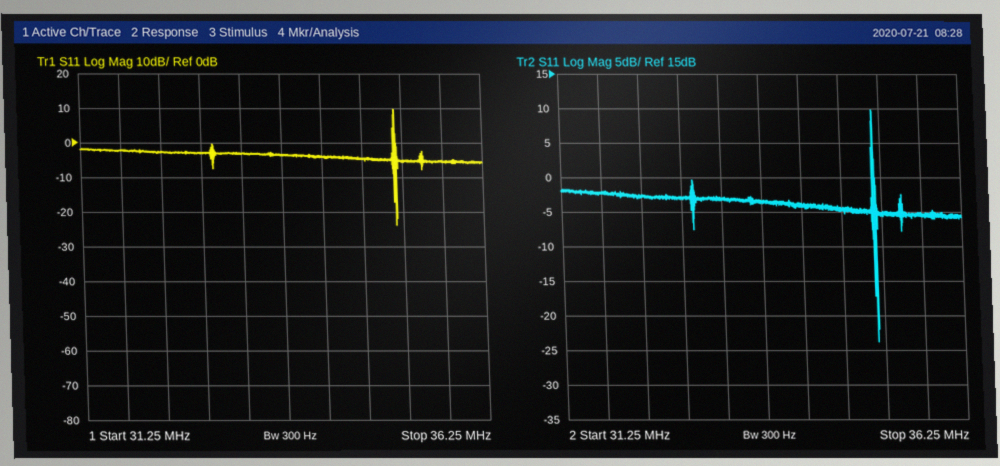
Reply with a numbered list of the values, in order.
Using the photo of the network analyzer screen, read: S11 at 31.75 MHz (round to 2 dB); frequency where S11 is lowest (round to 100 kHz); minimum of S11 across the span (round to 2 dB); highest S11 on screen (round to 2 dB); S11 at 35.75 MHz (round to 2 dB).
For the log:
1. -2 dB
2. 35.2 MHz
3. -24 dB
4. 10 dB
5. -6 dB
